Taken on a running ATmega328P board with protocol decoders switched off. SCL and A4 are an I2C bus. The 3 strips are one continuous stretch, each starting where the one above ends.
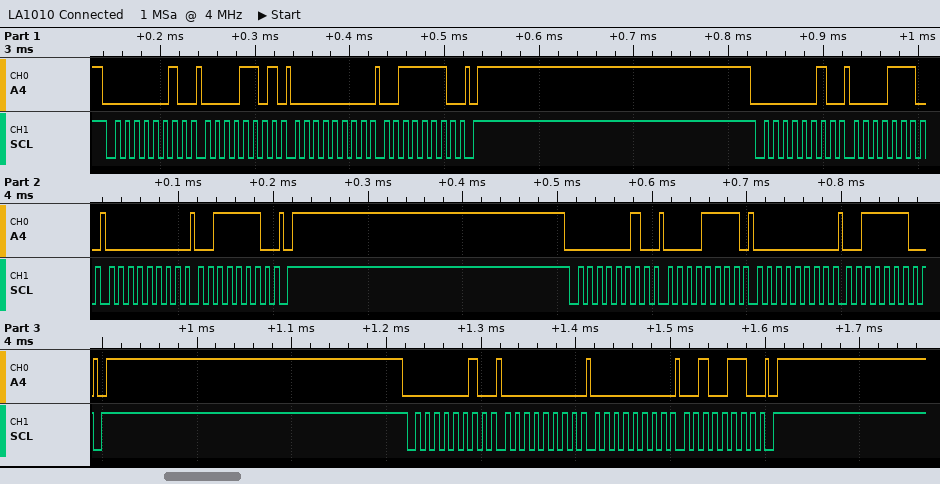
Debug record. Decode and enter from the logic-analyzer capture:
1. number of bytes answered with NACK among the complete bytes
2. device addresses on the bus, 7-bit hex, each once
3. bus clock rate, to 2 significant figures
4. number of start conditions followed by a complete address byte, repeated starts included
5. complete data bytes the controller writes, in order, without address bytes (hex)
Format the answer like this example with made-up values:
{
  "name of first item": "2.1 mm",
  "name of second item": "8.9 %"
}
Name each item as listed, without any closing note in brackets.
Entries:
{
  "number of bytes answered with NACK among the complete bytes": "0",
  "device addresses on the bus, 7-bit hex, each once": "0x01",
  "bus clock rate, to 2 significant figures": "100 kHz",
  "number of start conditions followed by a complete address byte, repeated starts included": "4",
  "complete data bytes the controller writes, in order, without address bytes": "0D 00 3E 0E 00 3E 0F 00 3E 00 00 26"
}
